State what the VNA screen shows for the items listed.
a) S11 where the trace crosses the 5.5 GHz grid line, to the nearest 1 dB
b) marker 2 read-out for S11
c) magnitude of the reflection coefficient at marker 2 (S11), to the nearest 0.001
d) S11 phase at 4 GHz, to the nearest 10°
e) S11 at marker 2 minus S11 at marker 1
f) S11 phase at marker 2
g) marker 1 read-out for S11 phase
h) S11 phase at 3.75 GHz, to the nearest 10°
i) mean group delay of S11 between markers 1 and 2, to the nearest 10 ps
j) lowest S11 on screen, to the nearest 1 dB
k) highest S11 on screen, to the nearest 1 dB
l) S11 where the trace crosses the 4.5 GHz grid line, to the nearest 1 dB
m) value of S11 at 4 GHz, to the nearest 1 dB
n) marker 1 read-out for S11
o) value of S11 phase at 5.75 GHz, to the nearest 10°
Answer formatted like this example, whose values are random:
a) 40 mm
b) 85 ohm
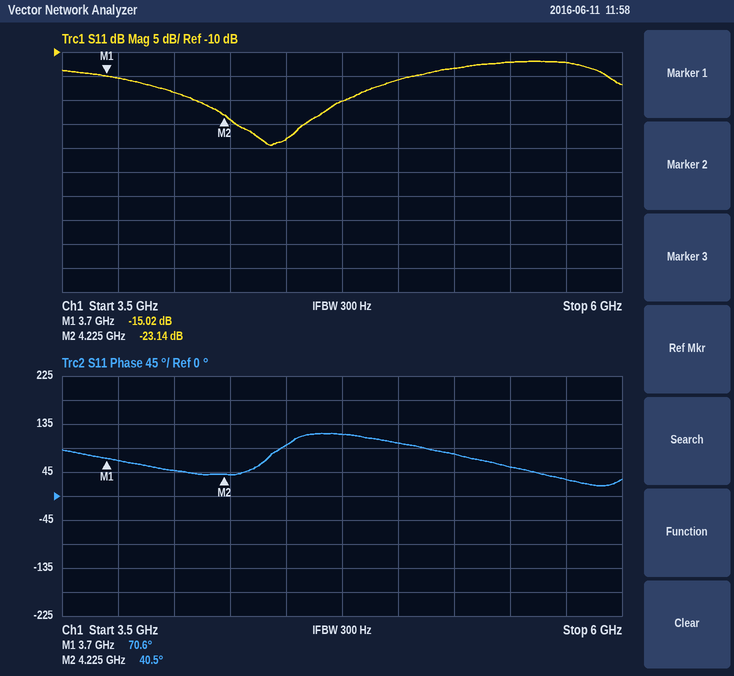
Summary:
a) -12 dB
b) -23.14 dB
c) 0.070
d) 50°
e) -8.12 dB
f) 40.5°
g) 70.6°
h) 70°
i) 160 ps
j) -29 dB
k) -12 dB
l) -28 dB
m) -18 dB
n) -15.02 dB
o) 30°
